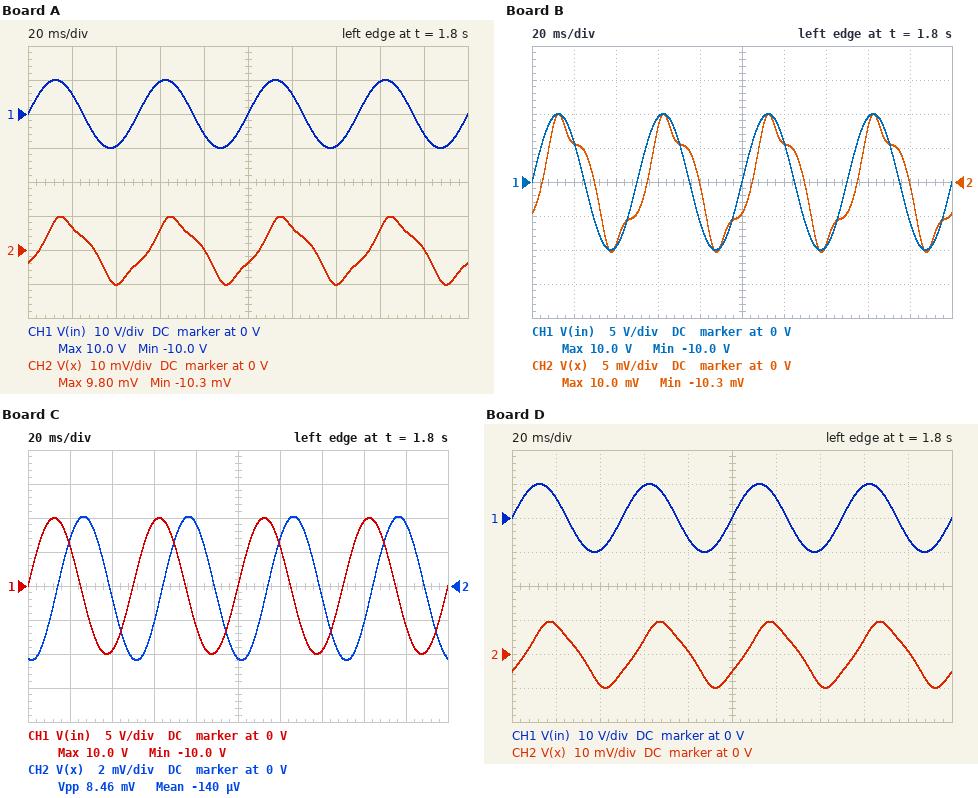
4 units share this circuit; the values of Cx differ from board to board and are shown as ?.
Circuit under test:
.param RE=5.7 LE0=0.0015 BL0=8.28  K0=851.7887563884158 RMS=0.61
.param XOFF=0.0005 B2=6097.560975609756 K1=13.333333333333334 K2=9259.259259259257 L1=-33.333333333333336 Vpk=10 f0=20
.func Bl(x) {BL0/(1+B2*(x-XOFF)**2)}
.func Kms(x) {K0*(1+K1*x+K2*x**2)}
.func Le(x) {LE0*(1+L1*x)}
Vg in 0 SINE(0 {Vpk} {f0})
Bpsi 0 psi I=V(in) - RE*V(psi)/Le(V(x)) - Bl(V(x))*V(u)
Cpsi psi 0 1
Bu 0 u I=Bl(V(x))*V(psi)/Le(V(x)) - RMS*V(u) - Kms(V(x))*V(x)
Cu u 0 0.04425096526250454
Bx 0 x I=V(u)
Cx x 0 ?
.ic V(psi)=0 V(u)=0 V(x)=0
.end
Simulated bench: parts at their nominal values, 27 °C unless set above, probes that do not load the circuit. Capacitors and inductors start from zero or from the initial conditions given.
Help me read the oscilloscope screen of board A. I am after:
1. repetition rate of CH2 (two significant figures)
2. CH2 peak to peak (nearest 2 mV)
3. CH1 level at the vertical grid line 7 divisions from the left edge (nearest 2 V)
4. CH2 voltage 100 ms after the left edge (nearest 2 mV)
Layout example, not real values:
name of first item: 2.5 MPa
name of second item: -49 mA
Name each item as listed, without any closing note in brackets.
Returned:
repetition rate of CH2: 20 Hz
CH2 peak to peak: 20 mV
CH1 level at the vertical grid line 7 divisions from the left edge: -10 V
CH2 voltage 100 ms after the left edge: -4 mV
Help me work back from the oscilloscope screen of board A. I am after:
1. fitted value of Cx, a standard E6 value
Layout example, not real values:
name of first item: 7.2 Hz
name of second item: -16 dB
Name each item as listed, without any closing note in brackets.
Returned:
fitted value of Cx, a standard E6 value: 470 mF
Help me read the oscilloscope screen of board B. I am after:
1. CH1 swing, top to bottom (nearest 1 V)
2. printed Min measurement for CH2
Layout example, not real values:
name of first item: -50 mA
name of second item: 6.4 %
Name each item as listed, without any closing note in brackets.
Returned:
CH1 swing, top to bottom: 20 V
printed Min measurement for CH2: -10.3 mV
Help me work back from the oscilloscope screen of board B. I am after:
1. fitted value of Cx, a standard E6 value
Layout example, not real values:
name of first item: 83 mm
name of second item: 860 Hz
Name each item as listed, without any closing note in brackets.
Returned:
fitted value of Cx, a standard E6 value: 330 mF
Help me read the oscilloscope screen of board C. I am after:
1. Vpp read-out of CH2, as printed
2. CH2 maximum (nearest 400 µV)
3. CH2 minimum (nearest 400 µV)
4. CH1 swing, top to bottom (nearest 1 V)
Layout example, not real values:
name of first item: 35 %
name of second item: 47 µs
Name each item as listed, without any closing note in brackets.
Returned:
Vpp read-out of CH2, as printed: 8.46 mV
CH2 maximum: 4.0 mV
CH2 minimum: -4.4 mV
CH1 swing, top to bottom: 20 V
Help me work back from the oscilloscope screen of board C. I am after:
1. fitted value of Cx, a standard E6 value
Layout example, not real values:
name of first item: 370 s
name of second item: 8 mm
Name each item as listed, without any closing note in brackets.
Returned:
fitted value of Cx, a standard E6 value: 2.2 F
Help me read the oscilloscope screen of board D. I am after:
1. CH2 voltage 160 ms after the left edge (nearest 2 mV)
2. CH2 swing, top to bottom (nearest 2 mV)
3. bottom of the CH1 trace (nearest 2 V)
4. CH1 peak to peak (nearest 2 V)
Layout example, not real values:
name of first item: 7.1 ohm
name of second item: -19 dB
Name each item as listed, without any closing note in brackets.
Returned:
CH2 voltage 160 ms after the left edge: 4 mV
CH2 swing, top to bottom: 20 mV
bottom of the CH1 trace: -10 V
CH1 peak to peak: 20 V
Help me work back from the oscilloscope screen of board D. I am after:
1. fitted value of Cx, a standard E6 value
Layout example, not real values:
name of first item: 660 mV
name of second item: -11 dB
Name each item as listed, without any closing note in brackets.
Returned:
fitted value of Cx, a standard E6 value: 680 mF
